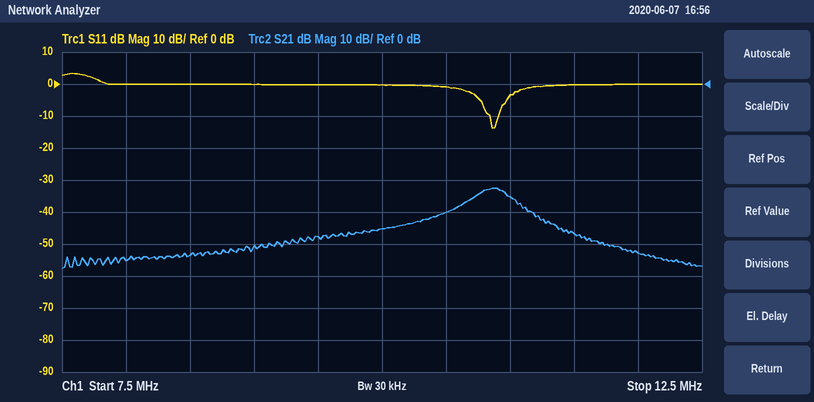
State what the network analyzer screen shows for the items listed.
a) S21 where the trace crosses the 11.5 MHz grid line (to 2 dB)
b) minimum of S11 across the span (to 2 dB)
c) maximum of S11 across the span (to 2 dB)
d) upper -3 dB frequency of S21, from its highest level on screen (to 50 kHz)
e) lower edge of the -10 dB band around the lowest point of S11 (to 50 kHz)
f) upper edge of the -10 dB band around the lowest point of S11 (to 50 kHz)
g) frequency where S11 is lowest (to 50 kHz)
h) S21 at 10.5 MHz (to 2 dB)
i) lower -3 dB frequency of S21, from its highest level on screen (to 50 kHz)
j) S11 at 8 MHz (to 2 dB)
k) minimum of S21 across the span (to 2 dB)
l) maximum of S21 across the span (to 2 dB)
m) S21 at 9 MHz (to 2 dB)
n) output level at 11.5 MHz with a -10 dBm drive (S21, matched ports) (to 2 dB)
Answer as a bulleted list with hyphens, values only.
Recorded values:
- -46 dB
- -14 dB
- 4 dB
- 11.00 MHz
- 10.85 MHz
- 10.90 MHz
- 10.85 MHz
- -40 dB
- 10.70 MHz
- 0 dB
- -58 dB
- -32 dB
- -50 dB
- -56 dBm
